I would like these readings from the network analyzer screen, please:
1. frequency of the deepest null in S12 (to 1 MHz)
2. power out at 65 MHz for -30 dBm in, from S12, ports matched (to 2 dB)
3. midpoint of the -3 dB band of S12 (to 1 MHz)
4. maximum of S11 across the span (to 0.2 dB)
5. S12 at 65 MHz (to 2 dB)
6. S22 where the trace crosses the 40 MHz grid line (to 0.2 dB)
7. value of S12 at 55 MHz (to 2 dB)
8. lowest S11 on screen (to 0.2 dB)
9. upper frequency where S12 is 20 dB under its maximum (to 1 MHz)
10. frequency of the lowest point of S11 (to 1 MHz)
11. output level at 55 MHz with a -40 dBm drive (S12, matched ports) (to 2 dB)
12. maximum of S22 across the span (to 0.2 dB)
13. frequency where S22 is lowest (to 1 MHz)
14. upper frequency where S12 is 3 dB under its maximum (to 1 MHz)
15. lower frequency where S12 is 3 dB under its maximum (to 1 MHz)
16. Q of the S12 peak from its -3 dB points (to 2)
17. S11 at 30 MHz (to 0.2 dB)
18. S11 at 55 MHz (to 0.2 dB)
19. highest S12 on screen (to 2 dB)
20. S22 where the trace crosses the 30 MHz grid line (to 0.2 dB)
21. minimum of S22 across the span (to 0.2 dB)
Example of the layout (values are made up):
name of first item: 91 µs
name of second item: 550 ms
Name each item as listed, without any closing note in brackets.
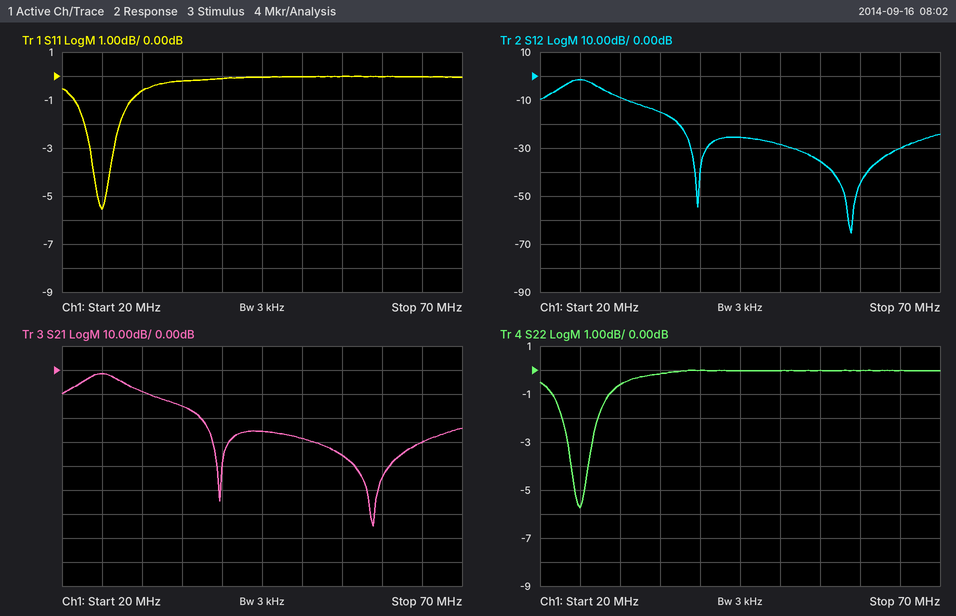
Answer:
frequency of the deepest null in S12: 59 MHz
power out at 65 MHz for -30 dBm in, from S12, ports matched: -60 dBm
midpoint of the -3 dB band of S12: 25 MHz
maximum of S11 across the span: 0.0 dB
S12 at 65 MHz: -30 dB
S22 where the trace crosses the 40 MHz grid line: 0.0 dB
value of S12 at 55 MHz: -36 dB
lowest S11 on screen: -5.6 dB
upper frequency where S12 is 20 dB under its maximum: 38 MHz
frequency of the lowest point of S11: 25 MHz
output level at 55 MHz with a -40 dBm drive (S12, matched ports): -76 dBm
maximum of S22 across the span: 0.0 dB
frequency where S22 is lowest: 25 MHz
upper frequency where S12 is 3 dB under its maximum: 27 MHz
lower frequency where S12 is 3 dB under its maximum: 23 MHz
Q of the S12 peak from its -3 dB points: 6
S11 at 30 MHz: -0.6 dB
S11 at 55 MHz: 0.0 dB
highest S12 on screen: -2 dB
S22 where the trace crosses the 30 MHz grid line: -0.6 dB
minimum of S22 across the span: -5.8 dB
